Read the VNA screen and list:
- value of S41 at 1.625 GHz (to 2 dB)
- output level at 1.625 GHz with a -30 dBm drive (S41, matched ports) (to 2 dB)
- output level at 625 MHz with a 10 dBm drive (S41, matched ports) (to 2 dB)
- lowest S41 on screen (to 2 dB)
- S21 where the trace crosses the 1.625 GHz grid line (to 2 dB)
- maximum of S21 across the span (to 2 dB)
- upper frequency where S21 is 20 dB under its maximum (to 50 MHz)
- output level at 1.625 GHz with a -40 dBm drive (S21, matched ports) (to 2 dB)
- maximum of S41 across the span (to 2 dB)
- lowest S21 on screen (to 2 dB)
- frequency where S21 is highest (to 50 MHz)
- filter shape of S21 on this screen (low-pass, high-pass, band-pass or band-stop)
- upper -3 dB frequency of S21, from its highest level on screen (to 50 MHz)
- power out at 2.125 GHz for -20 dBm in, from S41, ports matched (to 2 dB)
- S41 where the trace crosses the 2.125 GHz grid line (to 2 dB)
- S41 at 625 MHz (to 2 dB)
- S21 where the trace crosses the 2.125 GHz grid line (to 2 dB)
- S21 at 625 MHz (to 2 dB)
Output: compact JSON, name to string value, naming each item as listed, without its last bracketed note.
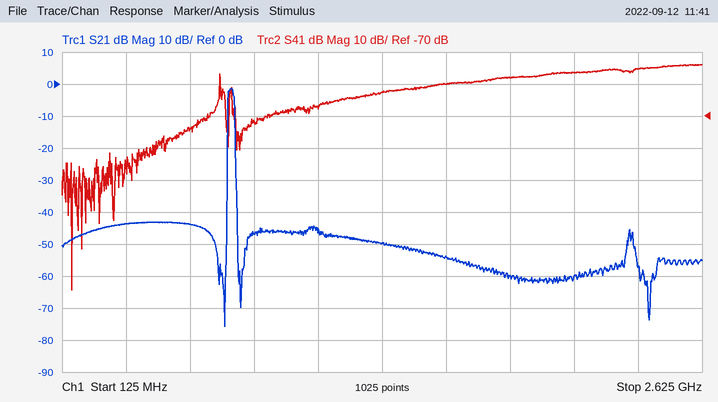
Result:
{"value of S41 at 1.625 GHz": "-60 dB", "output level at 1.625 GHz with a -30 dBm drive (S41, matched ports)": "-90 dBm", "output level at 625 MHz with a 10 dBm drive (S41, matched ports)": "-64 dBm", "lowest S41 on screen": "-124 dB", "S21 where the trace crosses the 1.625 GHz grid line": "-54 dB", "maximum of S21 across the span": "-2 dB", "upper frequency where S21 is 20 dB under its maximum": "800 MHz", "output level at 1.625 GHz with a -40 dBm drive (S21, matched ports)": "-94 dBm", "maximum of S41 across the span": "-54 dB", "lowest S21 on screen": "-76 dB", "frequency where S21 is highest": "800 MHz", "filter shape of S21 on this screen": "band-pass", "upper -3 dB frequency of S21, from its highest level on screen": "800 MHz", "power out at 2.125 GHz for -20 dBm in, from S41, ports matched": "-76 dBm", "S41 where the trace crosses the 2.125 GHz grid line": "-56 dB", "S41 at 625 MHz": "-74 dB", "S21 where the trace crosses the 2.125 GHz grid line": "-60 dB", "S21 at 625 MHz": "-44 dB"}
